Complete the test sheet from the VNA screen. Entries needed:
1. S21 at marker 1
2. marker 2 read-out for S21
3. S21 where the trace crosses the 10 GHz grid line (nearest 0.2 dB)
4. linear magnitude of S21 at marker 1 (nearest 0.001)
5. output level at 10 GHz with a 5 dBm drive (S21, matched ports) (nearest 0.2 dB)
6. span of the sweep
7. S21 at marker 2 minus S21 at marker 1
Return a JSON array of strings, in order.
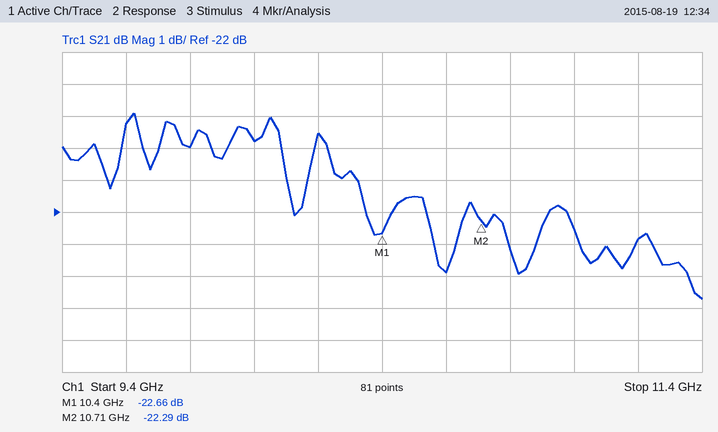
["-22.66 dB", "-22.29 dB", "-19.8 dB", "0.074", "-14.8 dBm", "2 GHz", "0.37 dB"]
